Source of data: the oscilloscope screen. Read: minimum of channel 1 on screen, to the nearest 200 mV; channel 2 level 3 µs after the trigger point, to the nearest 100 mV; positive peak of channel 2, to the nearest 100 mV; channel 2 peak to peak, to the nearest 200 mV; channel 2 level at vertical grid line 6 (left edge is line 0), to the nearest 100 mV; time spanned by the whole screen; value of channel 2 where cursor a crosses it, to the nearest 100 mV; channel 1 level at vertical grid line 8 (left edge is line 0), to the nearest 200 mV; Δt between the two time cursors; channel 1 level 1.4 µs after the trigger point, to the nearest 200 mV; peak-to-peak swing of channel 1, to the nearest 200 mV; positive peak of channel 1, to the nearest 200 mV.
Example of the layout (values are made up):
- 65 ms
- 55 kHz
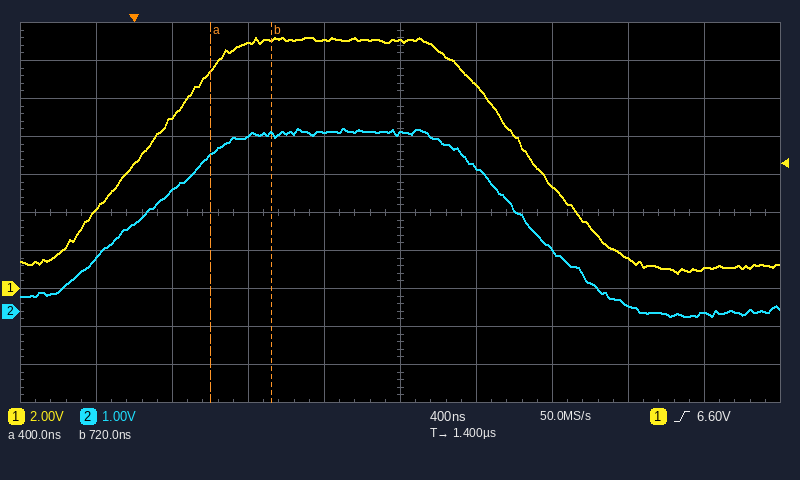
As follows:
- 800 mV
- 0.0 V
- 4.8 V
- 5.0 V
- 3.8 V
- 4 µs
- 4.1 V
- 1.6 V
- 320 ns
- 13.0 V
- 12.4 V
- 13.2 V
